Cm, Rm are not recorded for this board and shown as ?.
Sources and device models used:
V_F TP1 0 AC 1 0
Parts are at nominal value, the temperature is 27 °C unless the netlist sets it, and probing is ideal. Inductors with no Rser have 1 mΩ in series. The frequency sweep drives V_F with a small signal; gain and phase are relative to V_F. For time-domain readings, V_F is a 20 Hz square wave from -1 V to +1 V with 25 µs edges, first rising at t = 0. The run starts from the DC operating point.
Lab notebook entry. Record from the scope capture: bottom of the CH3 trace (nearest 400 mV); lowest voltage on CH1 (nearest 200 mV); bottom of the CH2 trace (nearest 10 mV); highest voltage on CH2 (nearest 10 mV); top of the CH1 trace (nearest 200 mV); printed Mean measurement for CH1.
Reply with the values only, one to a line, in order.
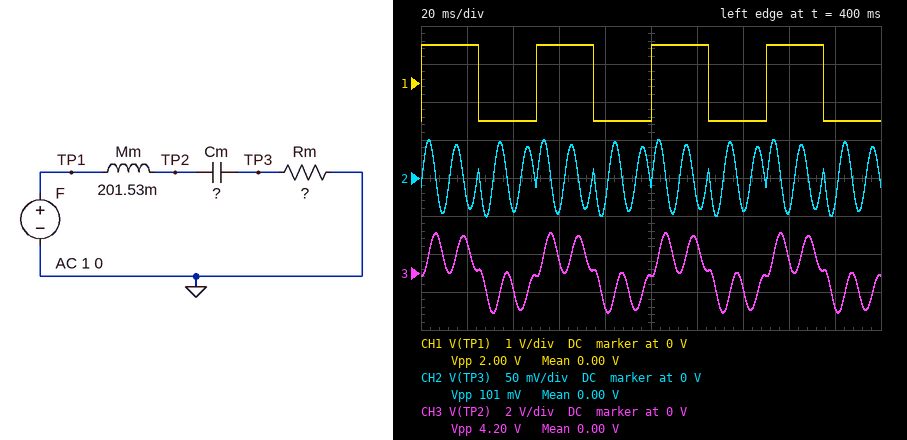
-2.0 V
-1.0 V
-50 mV
50 mV
1.0 V
0.00 V
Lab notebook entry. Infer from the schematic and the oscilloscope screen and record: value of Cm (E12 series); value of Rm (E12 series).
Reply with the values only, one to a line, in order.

18 µF
4.7 Ω
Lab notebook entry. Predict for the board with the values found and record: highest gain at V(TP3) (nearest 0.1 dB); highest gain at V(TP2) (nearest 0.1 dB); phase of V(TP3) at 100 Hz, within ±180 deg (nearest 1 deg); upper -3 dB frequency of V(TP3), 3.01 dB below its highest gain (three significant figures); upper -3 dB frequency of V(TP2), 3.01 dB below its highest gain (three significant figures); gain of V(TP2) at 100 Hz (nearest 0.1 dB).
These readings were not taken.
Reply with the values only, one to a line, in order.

0 dB
27.1 dB
-83 deg
85.4 Hz
85.4 Hz
7.2 dB
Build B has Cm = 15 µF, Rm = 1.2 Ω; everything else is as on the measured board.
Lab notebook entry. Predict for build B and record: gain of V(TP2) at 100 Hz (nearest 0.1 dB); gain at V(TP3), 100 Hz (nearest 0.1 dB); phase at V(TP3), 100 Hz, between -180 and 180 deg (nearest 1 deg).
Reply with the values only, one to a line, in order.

14.3 dB
-24.7 dB
-87 deg
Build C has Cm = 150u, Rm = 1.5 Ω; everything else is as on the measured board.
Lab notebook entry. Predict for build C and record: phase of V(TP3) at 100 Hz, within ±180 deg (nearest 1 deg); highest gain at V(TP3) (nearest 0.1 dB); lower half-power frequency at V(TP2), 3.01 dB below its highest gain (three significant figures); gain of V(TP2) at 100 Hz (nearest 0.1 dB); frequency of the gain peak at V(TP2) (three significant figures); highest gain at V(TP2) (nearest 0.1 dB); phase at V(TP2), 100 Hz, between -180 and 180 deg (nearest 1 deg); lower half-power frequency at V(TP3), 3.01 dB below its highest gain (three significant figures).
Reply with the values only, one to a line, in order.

-89 deg
0 dB
28.3 Hz
-20.7 dB
28.9 Hz
27.8 dB
-171 deg
28.4 Hz
